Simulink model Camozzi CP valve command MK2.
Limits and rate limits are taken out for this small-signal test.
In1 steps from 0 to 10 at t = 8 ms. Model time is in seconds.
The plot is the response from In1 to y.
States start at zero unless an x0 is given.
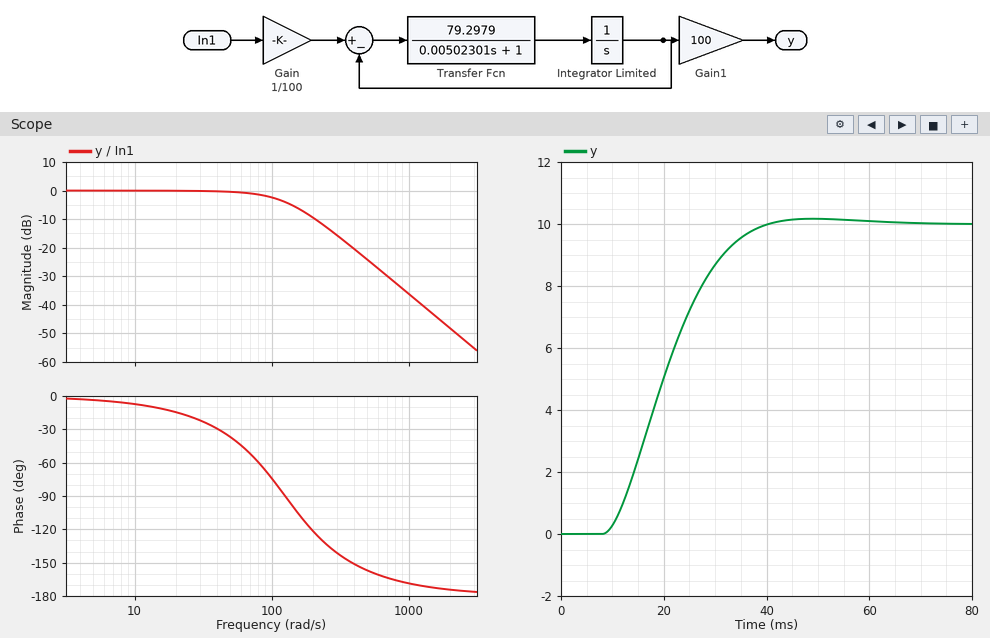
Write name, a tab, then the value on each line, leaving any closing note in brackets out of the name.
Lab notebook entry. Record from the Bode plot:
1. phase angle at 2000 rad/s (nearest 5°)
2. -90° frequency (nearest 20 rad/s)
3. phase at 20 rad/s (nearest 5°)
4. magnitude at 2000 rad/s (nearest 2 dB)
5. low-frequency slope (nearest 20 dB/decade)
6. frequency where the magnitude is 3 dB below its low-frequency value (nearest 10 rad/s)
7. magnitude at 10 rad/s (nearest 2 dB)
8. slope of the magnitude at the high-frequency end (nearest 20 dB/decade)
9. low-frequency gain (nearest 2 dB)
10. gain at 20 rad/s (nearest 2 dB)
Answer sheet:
phase angle at 2000 rad/s	-175°
-90° frequency	120 rad/s
phase at 20 rad/s	-15°
magnitude at 2000 rad/s	-48 dB
low-frequency slope	0 dB/decade
frequency where the magnitude is 3 dB below its low-frequency value	110 rad/s
magnitude at 10 rad/s	0 dB
slope of the magnitude at the high-frequency end	-40 dB/decade
low-frequency gain	0 dB
gain at 20 rad/s	0 dB
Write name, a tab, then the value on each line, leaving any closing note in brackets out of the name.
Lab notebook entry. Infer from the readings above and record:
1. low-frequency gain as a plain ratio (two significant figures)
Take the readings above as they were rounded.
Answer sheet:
low-frequency gain as a plain ratio	1.0
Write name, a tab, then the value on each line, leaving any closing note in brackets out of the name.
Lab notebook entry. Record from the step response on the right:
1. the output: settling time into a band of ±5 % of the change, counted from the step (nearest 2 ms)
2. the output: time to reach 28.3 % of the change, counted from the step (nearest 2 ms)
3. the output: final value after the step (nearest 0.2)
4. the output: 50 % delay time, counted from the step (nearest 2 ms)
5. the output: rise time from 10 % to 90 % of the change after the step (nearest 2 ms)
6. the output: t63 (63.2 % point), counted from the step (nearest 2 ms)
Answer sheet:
the output: settling time into a band of ±5 % of the change, counted from the step	26 ms
the output: time to reach 28.3 % of the change, counted from the step	8 ms
the output: final value after the step	10.0
the output: 50 % delay time, counted from the step	12 ms
the output: rise time from 10 % to 90 % of the change after the step	20 ms
the output: t63 (63.2 % point), counted from the step	14 ms
